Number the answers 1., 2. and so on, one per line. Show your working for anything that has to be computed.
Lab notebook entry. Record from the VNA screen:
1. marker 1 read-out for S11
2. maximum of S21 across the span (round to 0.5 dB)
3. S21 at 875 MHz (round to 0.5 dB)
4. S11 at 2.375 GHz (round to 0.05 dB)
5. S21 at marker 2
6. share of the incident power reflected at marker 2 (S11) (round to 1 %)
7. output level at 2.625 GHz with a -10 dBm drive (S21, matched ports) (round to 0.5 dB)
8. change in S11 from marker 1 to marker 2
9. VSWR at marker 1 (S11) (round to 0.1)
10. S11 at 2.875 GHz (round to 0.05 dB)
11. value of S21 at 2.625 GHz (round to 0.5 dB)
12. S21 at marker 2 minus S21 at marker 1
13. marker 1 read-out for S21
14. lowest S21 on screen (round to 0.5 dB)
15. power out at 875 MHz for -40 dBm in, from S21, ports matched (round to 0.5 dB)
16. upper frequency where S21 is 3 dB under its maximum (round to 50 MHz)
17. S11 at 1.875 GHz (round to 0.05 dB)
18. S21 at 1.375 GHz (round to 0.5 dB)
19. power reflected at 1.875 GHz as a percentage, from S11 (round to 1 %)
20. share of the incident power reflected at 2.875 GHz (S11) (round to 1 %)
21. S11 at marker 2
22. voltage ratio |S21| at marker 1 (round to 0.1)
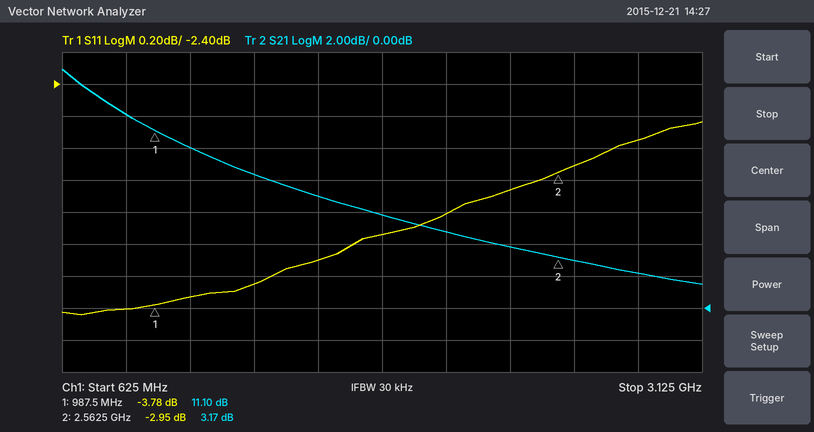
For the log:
1. -3.78 dB
2. 15.0 dB
3. 12.0 dB
4. -3.05 dB
5. 3.17 dB
6. 10^(-2.95/10) ≈ 51 %
7. -10 dBm + (3.0 dB) = -7.0 dBm
8. -2.95 − (-3.78) = 0.83 dB
9. (1 + 0.6471)/(1 − 0.6471) ≈ 4.7
10. -2.75 dB
11. 3.0 dB
12. 3.17 − (11.1) = -7.93 dB
13. 11.10 dB
14. 1.5 dB
15. -40 dBm + (12.0 dB) = -28.0 dBm
16. 900 MHz
17. -3.35 dB
18. 8.5 dB
19. 10^(-3.35/10) ≈ 46 %
20. 10^(-2.75/10) ≈ 53 %
21. -2.95 dB
22. 10^(11.1/20) ≈ 3.6
